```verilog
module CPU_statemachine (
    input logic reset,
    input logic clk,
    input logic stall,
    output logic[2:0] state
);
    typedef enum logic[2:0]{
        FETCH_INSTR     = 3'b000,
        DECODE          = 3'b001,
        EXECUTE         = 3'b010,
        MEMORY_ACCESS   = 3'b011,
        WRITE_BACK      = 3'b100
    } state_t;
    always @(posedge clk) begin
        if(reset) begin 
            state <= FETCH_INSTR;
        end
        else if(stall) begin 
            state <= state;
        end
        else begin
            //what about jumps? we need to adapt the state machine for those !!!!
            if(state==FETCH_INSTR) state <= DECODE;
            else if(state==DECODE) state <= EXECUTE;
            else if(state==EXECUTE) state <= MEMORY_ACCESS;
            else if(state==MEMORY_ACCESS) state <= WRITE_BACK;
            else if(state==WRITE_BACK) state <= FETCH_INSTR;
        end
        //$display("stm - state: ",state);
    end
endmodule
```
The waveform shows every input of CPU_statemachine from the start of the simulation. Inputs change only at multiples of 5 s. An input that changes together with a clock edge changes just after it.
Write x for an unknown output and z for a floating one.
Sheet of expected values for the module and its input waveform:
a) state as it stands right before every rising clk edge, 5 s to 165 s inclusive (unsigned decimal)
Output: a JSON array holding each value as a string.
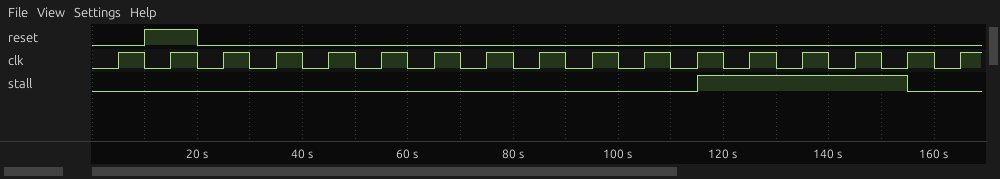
["x, x, 0, 1, 2, 3, 4, 0, 1, 2, 3, 4, 0, 0, 0, 0, 0"]
